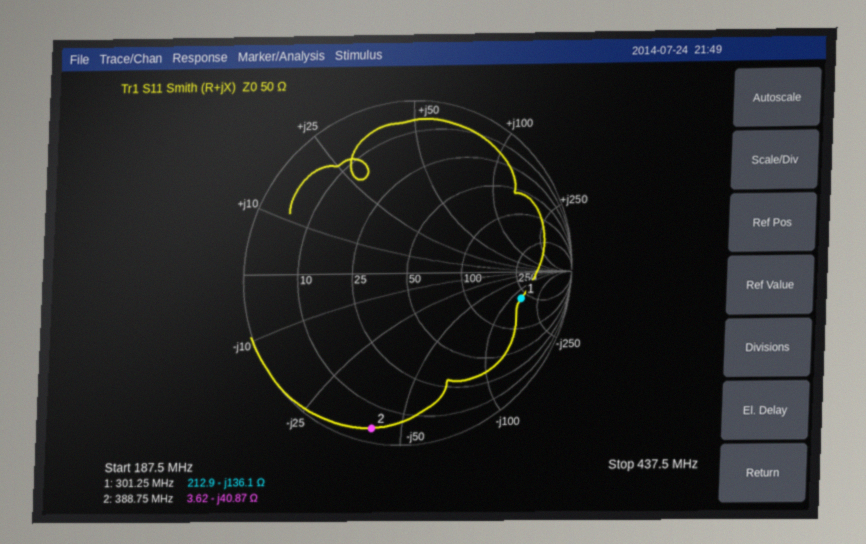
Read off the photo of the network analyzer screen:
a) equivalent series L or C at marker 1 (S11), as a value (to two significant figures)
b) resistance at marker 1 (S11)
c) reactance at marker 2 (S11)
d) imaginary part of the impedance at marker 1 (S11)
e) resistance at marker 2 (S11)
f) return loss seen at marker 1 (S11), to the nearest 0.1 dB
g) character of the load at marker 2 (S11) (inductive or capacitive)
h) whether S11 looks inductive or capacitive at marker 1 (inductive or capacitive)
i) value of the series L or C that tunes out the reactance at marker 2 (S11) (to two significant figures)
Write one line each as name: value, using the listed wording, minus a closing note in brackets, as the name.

equivalent series L or C at marker 1 (S11), as a value: 3.9 pF
resistance at marker 1: 212.9 Ω
reactance at marker 2: -40.87 Ω
imaginary part of the impedance at marker 1: -136.1 Ω
resistance at marker 2: 3.62 Ω
return loss seen at marker 1 (S11), to the nearest 0.1 dB: 2.9 dB
character of the load at marker 2 (S11): capacitive
whether S11 looks inductive or capacitive at marker 1: capacitive
value of the series L or C that tunes out the reactance at marker 2 (S11): 17 nH
